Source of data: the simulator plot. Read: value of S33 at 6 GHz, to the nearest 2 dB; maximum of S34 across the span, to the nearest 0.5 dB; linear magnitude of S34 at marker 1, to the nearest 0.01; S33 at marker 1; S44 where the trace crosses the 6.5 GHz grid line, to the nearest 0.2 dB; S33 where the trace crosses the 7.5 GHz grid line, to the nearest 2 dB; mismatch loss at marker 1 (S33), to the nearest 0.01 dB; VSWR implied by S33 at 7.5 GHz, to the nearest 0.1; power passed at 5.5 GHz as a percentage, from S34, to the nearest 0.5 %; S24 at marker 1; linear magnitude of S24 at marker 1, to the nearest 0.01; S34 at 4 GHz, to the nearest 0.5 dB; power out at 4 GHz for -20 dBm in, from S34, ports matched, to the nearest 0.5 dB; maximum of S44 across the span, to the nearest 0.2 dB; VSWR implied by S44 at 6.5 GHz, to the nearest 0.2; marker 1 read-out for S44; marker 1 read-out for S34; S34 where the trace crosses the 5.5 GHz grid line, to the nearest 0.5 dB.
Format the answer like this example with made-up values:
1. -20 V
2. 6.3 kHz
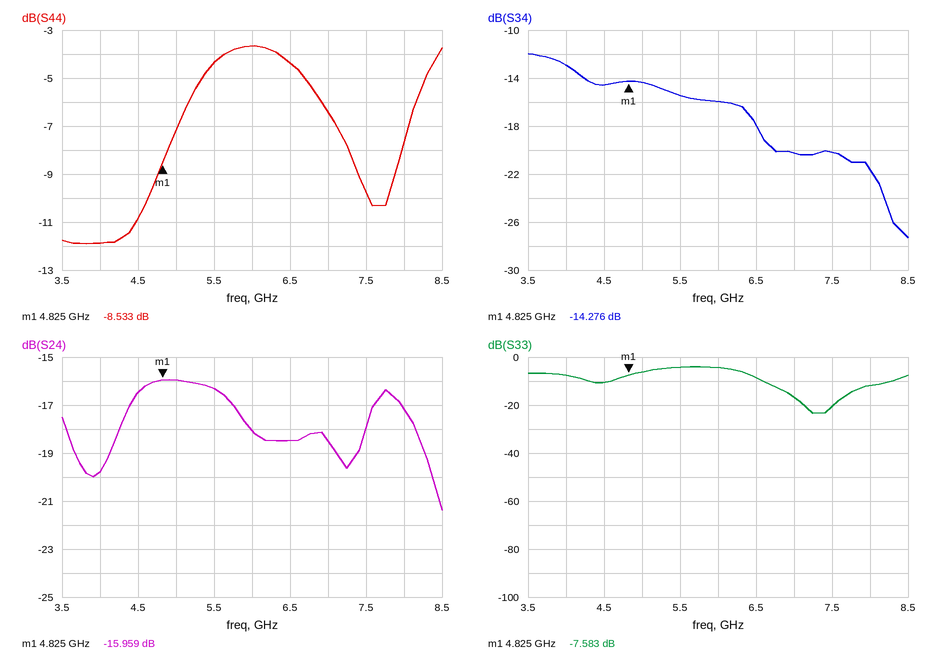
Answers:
1. -4 dB
2. -12.0 dB
3. 0.19
4. -7.583 dB
5. -4.4 dB
6. -20 dB
7. 0.83 dB
8. 1.2
9. 3.0 %
10. -15.959 dB
11. 0.16
12. -13.0 dB
13. -33.0 dBm
14. -3.6 dB
15. 4.0
16. -8.533 dB
17. -14.276 dB
18. -15.5 dB
